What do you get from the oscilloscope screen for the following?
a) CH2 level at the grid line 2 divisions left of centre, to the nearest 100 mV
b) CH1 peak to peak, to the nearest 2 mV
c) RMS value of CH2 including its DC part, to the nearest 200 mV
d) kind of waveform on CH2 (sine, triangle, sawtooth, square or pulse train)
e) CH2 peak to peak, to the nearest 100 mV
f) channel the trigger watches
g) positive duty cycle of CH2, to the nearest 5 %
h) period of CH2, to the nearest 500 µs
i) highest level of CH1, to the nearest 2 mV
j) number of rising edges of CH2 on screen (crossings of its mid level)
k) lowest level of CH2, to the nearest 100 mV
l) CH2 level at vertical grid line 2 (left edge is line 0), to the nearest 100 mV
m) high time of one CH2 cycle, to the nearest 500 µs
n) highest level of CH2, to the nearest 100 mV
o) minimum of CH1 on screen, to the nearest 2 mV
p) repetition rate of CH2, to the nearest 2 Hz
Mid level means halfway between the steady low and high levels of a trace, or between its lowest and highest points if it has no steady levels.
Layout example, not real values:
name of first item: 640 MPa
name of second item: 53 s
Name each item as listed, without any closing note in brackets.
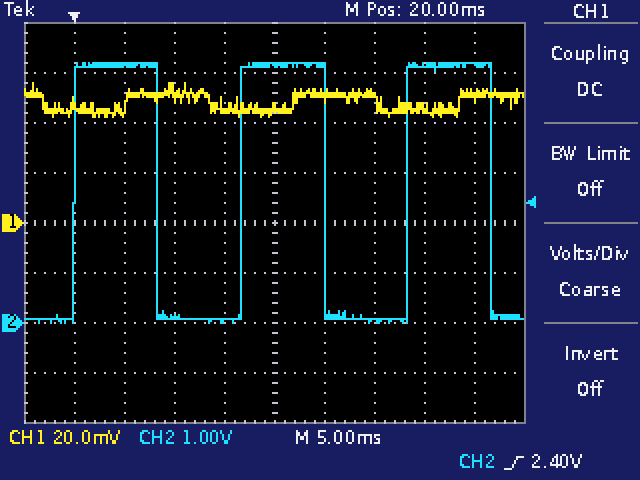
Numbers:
CH2 level at the grid line 2 divisions left of centre, to the nearest 100 mV: 100 mV
CH1 peak to peak, to the nearest 2 mV: 14 mV
RMS value of CH2 including its DC part, to the nearest 200 mV: 3.6 V
kind of waveform on CH2: square
CH2 peak to peak, to the nearest 100 mV: 5.2 V
channel the trigger watches: CH2
positive duty cycle of CH2, to the nearest 5 %: 50 %
period of CH2, to the nearest 500 µs: 16.5 ms
highest level of CH1, to the nearest 2 mV: 56 mV
number of rising edges of CH2 on screen: 3
lowest level of CH2, to the nearest 100 mV: 0.0 V
CH2 level at vertical grid line 2 (left edge is line 0), to the nearest 100 mV: 5.2 V
high time of one CH2 cycle, to the nearest 500 µs: 8.5 ms
highest level of CH2, to the nearest 100 mV: 5.2 V
minimum of CH1 on screen, to the nearest 2 mV: 42 mV
repetition rate of CH2, to the nearest 2 Hz: 60 Hz
